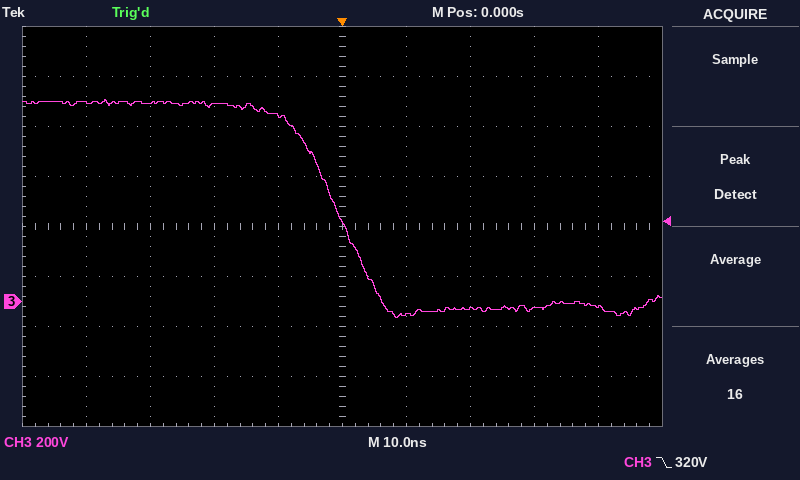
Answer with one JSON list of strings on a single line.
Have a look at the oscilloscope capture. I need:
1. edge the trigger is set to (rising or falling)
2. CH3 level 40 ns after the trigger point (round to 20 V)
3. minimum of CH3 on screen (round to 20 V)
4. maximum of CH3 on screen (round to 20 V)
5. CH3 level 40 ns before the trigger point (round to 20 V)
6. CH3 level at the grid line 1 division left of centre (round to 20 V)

["falling", "-20 V", "-60 V", "800 V", "800 V", "740 V"]
